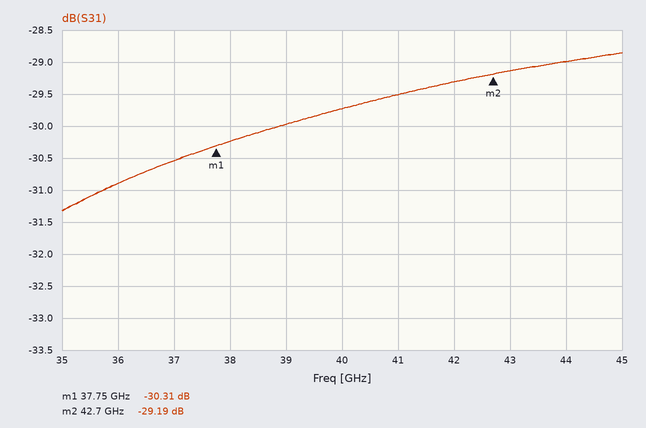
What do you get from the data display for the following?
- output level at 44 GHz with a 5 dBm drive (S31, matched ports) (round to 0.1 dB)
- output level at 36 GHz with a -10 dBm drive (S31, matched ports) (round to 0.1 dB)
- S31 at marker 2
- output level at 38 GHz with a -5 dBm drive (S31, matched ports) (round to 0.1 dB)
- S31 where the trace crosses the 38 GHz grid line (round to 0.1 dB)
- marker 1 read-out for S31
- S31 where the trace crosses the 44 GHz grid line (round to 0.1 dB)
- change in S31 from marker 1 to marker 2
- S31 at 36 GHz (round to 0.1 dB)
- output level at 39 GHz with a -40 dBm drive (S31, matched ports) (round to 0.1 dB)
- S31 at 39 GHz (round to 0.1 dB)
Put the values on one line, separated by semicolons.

-24.0 dBm; -40.9 dBm; -29.19 dB; -35.2 dBm; -30.2 dB; -30.31 dB; -29.0 dB; 1.12 dB; -30.9 dB; -70.0 dBm; -30.0 dB
